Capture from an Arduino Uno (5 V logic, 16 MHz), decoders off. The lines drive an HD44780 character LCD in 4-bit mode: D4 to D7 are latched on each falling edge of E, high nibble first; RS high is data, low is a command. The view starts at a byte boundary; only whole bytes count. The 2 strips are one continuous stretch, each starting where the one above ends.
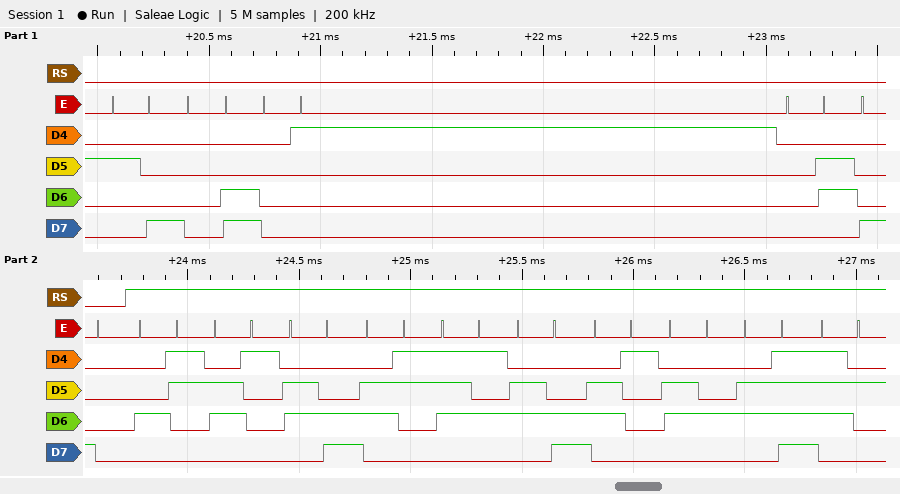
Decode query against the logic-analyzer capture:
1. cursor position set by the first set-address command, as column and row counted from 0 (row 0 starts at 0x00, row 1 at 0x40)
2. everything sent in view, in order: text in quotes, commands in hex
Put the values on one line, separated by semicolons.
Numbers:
column 0, row 0; 0x28 0x0C 0x01 0x06 0x80 "Calculador"
